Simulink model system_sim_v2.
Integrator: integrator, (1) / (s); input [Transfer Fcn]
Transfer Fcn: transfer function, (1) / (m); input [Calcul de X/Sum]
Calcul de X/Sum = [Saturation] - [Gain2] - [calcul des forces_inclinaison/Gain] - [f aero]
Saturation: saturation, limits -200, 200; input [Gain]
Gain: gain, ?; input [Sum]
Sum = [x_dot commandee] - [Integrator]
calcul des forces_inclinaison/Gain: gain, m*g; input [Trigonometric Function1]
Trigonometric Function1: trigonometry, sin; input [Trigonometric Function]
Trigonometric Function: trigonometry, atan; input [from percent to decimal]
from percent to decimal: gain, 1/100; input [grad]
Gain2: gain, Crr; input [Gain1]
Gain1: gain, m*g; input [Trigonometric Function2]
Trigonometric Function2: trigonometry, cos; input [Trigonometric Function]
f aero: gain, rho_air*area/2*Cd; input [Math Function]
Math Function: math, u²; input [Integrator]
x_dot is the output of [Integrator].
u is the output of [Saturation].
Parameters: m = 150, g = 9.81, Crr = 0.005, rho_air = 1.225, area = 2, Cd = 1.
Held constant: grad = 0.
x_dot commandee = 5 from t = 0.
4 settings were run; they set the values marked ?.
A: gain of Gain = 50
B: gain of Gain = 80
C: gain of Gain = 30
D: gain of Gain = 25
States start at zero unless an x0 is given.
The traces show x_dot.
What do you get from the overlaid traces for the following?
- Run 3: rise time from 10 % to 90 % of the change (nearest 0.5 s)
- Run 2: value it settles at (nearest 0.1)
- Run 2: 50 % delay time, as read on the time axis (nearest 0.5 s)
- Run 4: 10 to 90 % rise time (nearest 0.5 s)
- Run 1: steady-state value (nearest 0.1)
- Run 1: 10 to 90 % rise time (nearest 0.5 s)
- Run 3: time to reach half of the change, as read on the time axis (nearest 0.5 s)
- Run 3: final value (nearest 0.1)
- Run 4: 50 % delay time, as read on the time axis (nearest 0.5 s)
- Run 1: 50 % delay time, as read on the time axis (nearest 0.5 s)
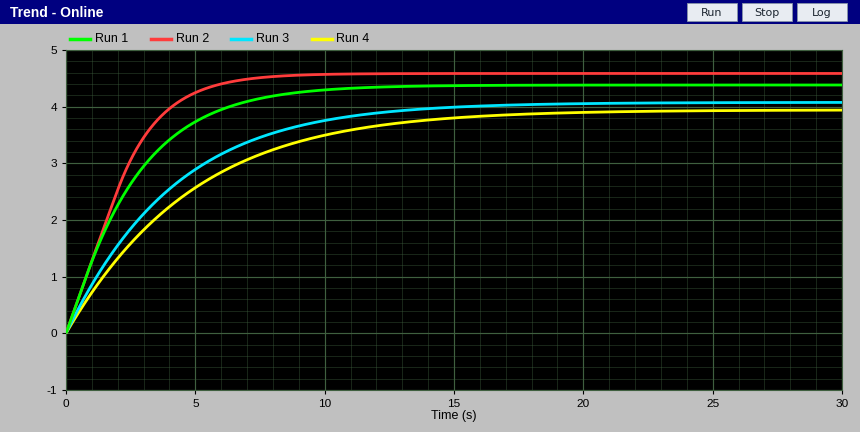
8.5 s
4.6
2.0 s
10.0 s
4.4
5.5 s
3.0 s
4.1
3.5 s
2.0 s
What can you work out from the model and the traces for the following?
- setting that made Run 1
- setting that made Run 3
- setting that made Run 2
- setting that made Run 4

A
C
B
D
